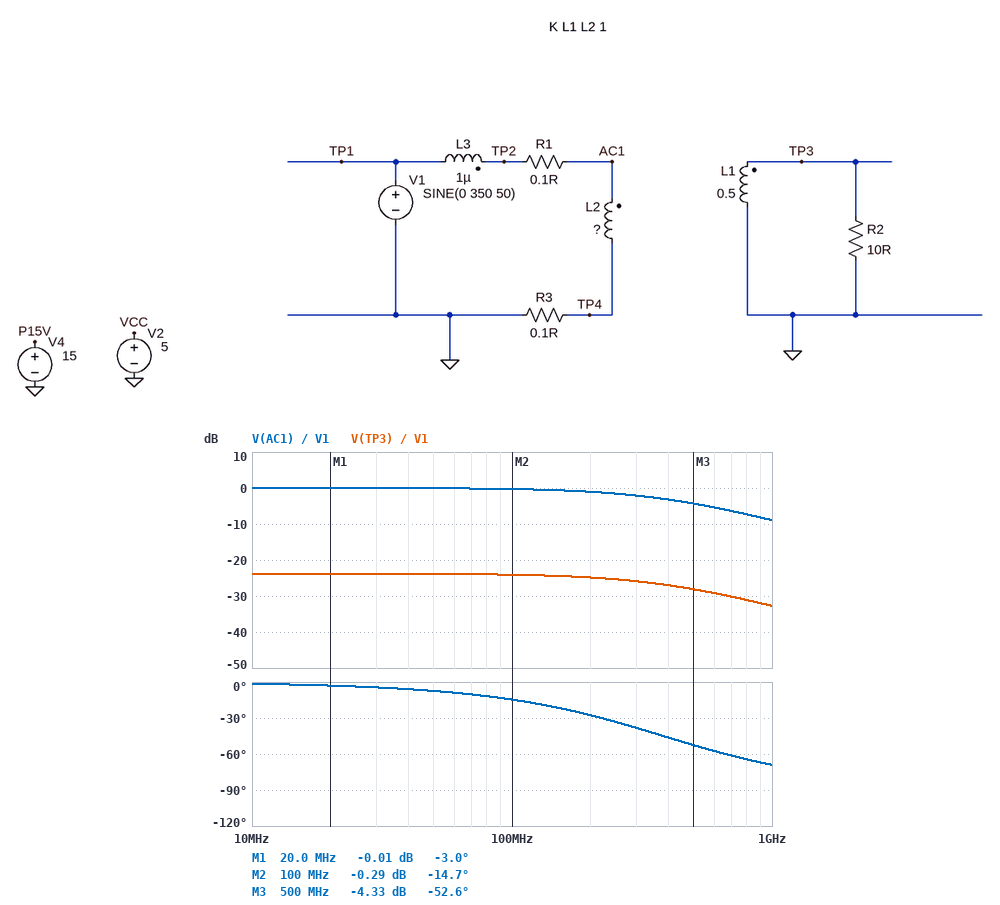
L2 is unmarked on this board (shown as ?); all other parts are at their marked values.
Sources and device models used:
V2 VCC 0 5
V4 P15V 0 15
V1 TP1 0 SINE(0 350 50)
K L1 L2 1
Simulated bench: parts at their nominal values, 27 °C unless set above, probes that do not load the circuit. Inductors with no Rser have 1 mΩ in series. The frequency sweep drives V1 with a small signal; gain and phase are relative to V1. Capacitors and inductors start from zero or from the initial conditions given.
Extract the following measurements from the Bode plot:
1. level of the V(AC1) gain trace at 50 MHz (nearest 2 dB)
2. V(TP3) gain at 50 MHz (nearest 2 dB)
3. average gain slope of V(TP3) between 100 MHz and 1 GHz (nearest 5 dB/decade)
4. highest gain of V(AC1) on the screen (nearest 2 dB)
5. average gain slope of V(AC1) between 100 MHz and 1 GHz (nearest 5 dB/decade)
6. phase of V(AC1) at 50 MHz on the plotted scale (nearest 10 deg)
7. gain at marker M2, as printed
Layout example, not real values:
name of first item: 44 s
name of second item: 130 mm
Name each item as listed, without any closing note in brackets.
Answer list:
level of the V(AC1) gain trace at 50 MHz: 0 dB
V(TP3) gain at 50 MHz: -24 dB
average gain slope of V(TP3) between 100 MHz and 1 GHz: -10 dB/decade
highest gain of V(AC1) on the screen: 0 dB
average gain slope of V(AC1) between 100 MHz and 1 GHz: -10 dB/decade
phase of V(AC1) at 50 MHz on the plotted scale: -10 deg
gain at marker M2, as printed: -0.29 dB
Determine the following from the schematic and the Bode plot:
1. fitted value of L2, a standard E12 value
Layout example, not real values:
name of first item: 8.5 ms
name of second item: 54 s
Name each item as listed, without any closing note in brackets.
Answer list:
fitted value of L2, a standard E12 value: 120 H
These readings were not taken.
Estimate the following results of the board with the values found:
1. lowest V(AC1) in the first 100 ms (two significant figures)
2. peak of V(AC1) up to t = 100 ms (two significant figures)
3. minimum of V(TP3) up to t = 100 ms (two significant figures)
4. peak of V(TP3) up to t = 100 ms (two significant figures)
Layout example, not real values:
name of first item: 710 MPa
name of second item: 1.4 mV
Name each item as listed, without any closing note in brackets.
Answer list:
lowest V(AC1) in the first 100 ms: -350 V
peak of V(AC1) up to t = 100 ms: 350 V
minimum of V(TP3) up to t = 100 ms: -23 V
peak of V(TP3) up to t = 100 ms: 23 V
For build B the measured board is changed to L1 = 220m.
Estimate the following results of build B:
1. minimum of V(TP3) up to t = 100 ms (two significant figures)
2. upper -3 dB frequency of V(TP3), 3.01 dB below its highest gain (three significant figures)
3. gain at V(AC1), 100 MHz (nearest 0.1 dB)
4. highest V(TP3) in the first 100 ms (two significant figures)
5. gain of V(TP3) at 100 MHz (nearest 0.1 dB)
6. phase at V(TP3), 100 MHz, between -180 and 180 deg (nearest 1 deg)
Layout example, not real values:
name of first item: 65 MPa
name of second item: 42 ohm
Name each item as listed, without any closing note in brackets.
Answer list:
minimum of V(TP3) up to t = 100 ms: -15 V
upper -3 dB frequency of V(TP3), 3.01 dB below its highest gain: 868 MHz
gain at V(AC1), 100 MHz: -0.1 dB
highest V(TP3) in the first 100 ms: 15 V
gain of V(TP3) at 100 MHz: -27.4 dB
phase at V(TP3), 100 MHz, between -180 and 180 deg: -7 deg
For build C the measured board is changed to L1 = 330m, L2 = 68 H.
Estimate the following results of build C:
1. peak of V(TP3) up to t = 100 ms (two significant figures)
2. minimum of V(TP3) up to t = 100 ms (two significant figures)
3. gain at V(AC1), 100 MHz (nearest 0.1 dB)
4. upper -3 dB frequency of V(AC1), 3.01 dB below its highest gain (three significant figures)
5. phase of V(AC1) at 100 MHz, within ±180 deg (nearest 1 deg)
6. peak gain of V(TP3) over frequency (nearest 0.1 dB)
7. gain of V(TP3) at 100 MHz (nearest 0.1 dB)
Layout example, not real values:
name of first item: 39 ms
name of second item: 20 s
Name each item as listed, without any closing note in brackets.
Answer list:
peak of V(TP3) up to t = 100 ms: 24 V
minimum of V(TP3) up to t = 100 ms: -24 V
gain at V(AC1), 100 MHz: -0.4 dB
upper -3 dB frequency of V(AC1), 3.01 dB below its highest gain: 328 MHz
phase of V(AC1) at 100 MHz, within ±180 deg: -17 deg
peak gain of V(TP3) over frequency: -23.1 dB
gain of V(TP3) at 100 MHz: -23.5 dB
